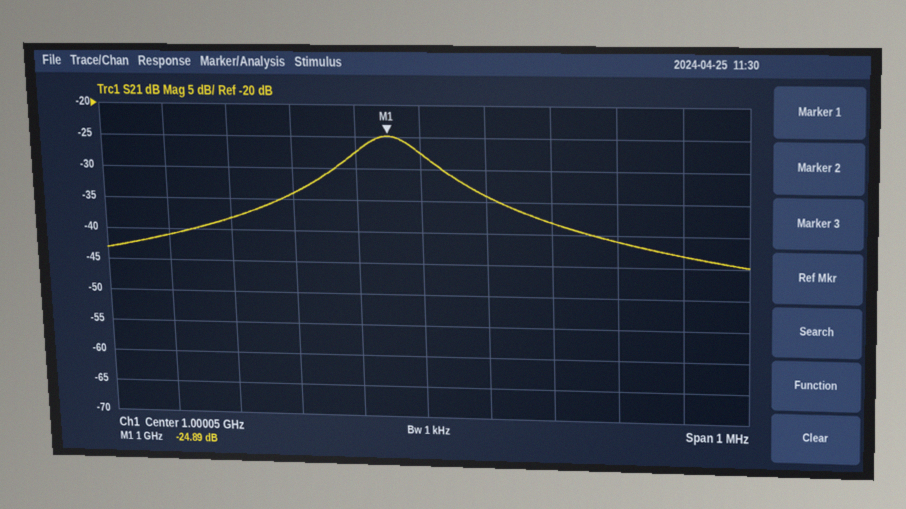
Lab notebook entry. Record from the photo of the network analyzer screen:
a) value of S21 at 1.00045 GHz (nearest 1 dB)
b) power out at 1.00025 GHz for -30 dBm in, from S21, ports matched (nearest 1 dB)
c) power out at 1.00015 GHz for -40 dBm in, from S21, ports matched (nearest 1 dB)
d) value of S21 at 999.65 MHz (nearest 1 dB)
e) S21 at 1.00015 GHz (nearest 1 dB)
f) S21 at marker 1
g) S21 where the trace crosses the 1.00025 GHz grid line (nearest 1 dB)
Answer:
-43 dB
-68 dBm
-74 dBm
-41 dB
-34 dB
-24.89 dB
-38 dB
